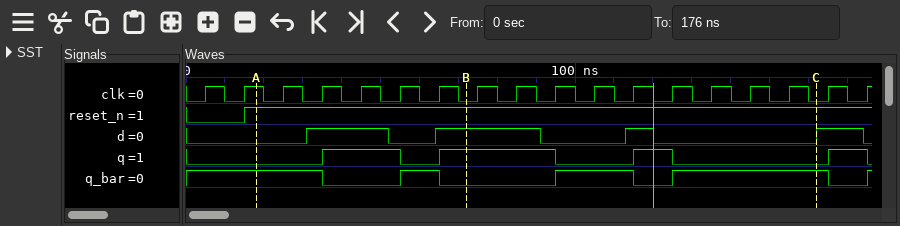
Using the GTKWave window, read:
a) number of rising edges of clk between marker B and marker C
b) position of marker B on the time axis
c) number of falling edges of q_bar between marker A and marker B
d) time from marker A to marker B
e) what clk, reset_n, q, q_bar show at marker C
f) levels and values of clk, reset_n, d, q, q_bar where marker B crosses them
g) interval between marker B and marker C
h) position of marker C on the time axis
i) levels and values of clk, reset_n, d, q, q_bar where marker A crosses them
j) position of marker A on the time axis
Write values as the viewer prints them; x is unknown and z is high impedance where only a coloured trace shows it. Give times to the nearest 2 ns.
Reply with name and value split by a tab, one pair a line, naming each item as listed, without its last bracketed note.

number of rising edges of clk between marker B and marker C	9
position of marker B on the time axis	72 ns
number of falling edges of q_bar between marker A and marker B	2
time from marker A to marker B	54 ns
what clk, reset_n, q, q_bar show at marker C	clk=0, reset_n=1, q=0, q_bar=1
levels and values of clk, reset_n, d, q, q_bar where marker B crosses them	clk=0, reset_n=1, d=1, q=1, q_bar=0
interval between marker B and marker C	90 ns
position of marker C on the time axis	162 ns
levels and values of clk, reset_n, d, q, q_bar where marker A crosses them	clk=1, reset_n=1, d=0, q=0, q_bar=1
position of marker A on the time axis	18 ns
